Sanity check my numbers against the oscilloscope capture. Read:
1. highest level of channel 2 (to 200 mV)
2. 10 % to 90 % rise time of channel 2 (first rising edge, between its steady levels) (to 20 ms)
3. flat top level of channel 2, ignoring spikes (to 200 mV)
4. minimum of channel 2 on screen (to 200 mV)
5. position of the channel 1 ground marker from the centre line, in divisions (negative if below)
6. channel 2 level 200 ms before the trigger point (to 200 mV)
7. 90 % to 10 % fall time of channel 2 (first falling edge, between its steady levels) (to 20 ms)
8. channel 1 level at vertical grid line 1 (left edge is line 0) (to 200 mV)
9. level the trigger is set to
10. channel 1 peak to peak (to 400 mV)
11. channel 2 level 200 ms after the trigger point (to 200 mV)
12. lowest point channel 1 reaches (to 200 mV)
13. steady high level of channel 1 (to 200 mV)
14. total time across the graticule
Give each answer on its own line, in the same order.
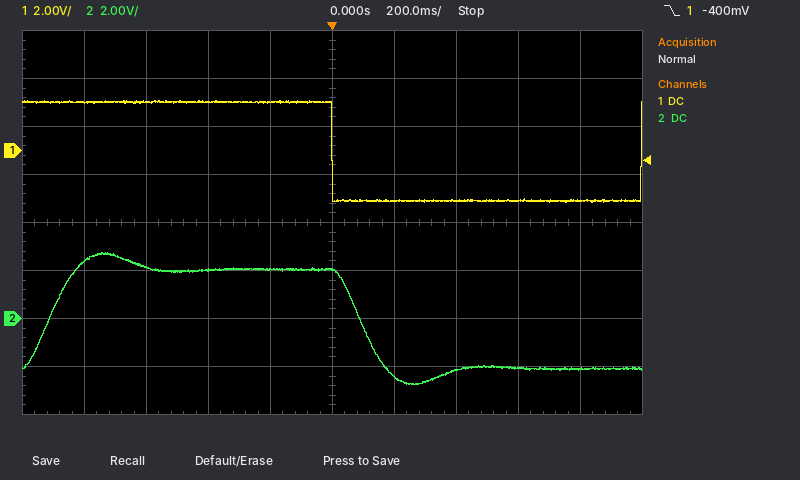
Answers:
2.8 V
120 ms
2.0 V
-2.8 V
+1.5 div
2.0 V
120 ms
2.0 V
-400 mV
4.4 V
-2.4 V
-2.2 V
2.0 V
2 s
